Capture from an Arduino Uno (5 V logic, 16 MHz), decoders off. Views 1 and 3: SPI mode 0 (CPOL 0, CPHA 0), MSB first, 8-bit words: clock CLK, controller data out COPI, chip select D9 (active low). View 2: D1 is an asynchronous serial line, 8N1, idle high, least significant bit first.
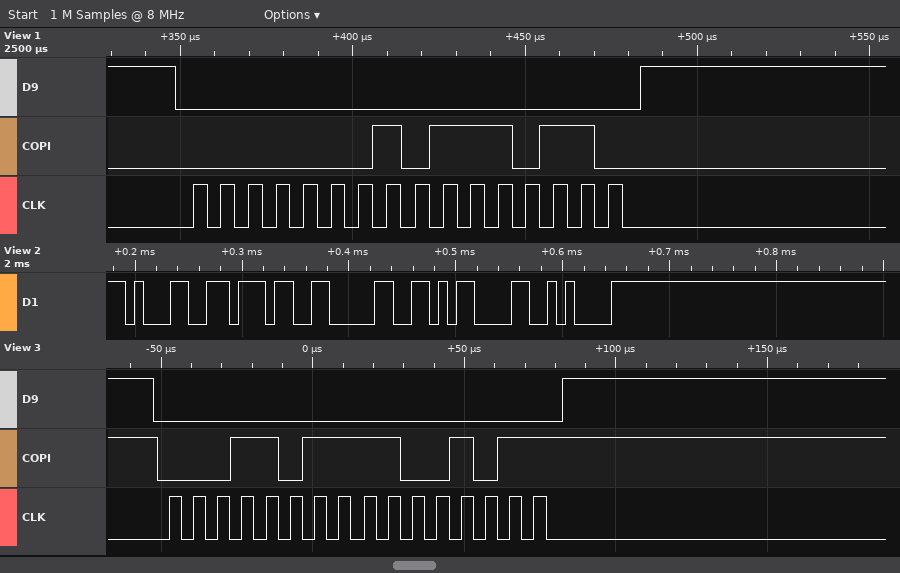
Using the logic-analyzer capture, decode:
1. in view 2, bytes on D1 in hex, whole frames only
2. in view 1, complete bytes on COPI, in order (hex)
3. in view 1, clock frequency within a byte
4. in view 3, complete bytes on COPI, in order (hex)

31 37 30 0D 0A
0x01 0x76
125 kHz
1B CB
